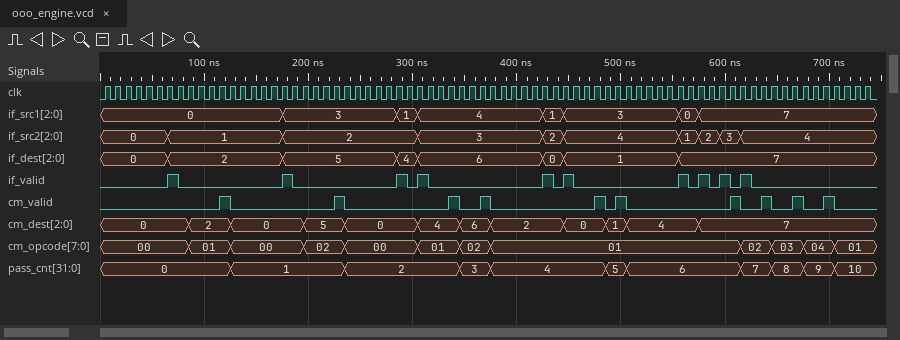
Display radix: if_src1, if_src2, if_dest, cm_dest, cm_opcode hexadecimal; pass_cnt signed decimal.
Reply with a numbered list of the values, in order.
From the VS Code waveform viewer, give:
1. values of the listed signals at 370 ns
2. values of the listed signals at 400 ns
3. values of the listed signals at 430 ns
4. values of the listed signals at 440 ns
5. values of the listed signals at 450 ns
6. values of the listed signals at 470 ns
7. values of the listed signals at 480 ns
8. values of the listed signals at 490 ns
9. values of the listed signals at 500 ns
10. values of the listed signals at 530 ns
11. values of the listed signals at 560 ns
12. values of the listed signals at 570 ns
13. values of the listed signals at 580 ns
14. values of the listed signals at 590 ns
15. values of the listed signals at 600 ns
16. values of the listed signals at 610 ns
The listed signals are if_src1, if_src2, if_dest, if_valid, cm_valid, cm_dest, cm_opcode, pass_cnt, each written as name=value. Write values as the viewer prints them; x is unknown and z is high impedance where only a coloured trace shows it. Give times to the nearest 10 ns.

1. if_src1=4, if_src2=3, if_dest=6, if_valid=0, cm_valid=1, cm_dest=6, cm_opcode=02, pass_cnt=3
2. if_src1=4, if_src2=3, if_dest=6, if_valid=0, cm_valid=0, cm_dest=2, cm_opcode=01, pass_cnt=4
3. if_src1=1, if_src2=2, if_dest=0, if_valid=1, cm_valid=0, cm_dest=2, cm_opcode=01, pass_cnt=4
4. if_src1=1, if_src2=2, if_dest=0, if_valid=0, cm_valid=0, cm_dest=2, cm_opcode=01, pass_cnt=4
5. if_src1=3, if_src2=4, if_dest=1, if_valid=1, cm_valid=0, cm_dest=0, cm_opcode=01, pass_cnt=4
6. if_src1=3, if_src2=4, if_dest=1, if_valid=0, cm_valid=0, cm_dest=0, cm_opcode=01, pass_cnt=4
7. if_src1=3, if_src2=4, if_dest=1, if_valid=0, cm_valid=1, cm_dest=0, cm_opcode=01, pass_cnt=4
8. if_src1=3, if_src2=4, if_dest=1, if_valid=0, cm_valid=0, cm_dest=1, cm_opcode=01, pass_cnt=5
9. if_src1=3, if_src2=4, if_dest=1, if_valid=0, cm_valid=1, cm_dest=1, cm_opcode=01, pass_cnt=5
10. if_src1=3, if_src2=4, if_dest=1, if_valid=0, cm_valid=0, cm_dest=4, cm_opcode=01, pass_cnt=6
11. if_src1=0, if_src2=1, if_dest=7, if_valid=1, cm_valid=0, cm_dest=4, cm_opcode=01, pass_cnt=6
12. if_src1=0, if_src2=1, if_dest=7, if_valid=0, cm_valid=0, cm_dest=4, cm_opcode=01, pass_cnt=6
13. if_src1=7, if_src2=2, if_dest=7, if_valid=1, cm_valid=0, cm_dest=7, cm_opcode=01, pass_cnt=6
14. if_src1=7, if_src2=2, if_dest=7, if_valid=0, cm_valid=0, cm_dest=7, cm_opcode=01, pass_cnt=6
15. if_src1=7, if_src2=3, if_dest=7, if_valid=1, cm_valid=0, cm_dest=7, cm_opcode=01, pass_cnt=6
16. if_src1=7, if_src2=3, if_dest=7, if_valid=0, cm_valid=1, cm_dest=7, cm_opcode=01, pass_cnt=6
